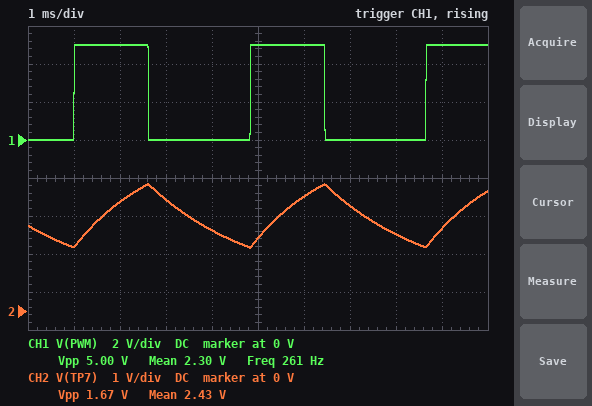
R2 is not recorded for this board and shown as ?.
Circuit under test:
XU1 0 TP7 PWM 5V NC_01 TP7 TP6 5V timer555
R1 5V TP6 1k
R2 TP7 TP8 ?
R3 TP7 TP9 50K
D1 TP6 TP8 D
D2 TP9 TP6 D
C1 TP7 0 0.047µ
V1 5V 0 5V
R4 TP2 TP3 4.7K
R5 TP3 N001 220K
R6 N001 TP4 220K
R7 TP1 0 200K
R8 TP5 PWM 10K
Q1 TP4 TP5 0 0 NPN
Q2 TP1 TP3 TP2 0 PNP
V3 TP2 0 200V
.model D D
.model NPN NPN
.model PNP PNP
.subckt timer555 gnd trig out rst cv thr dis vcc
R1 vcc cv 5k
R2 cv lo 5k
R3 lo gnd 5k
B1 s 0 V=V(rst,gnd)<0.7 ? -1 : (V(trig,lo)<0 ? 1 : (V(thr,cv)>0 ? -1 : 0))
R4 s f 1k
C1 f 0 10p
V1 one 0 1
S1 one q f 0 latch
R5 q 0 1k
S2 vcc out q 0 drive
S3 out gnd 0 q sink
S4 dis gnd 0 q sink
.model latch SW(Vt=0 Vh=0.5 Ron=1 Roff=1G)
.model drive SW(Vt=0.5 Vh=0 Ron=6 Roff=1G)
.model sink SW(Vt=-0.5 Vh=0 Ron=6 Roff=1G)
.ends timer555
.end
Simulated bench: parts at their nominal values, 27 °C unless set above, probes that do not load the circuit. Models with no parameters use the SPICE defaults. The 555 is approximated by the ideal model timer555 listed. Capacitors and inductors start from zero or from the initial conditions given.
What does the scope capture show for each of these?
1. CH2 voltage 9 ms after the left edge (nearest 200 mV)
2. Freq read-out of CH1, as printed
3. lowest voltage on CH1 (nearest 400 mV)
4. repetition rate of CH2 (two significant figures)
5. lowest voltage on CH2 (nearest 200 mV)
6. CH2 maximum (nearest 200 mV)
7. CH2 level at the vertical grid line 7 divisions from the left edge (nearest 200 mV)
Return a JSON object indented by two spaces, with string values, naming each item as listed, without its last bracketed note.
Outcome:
{
  "CH2 voltage 9 ms after the left edge": "2.2 V",
  "Freq read-out of CH1, as printed": "261 Hz",
  "lowest voltage on CH1": "0 V",
  "repetition rate of CH2": "260 Hz",
  "lowest voltage on CH2": "1.6 V",
  "CH2 maximum": "3.4 V",
  "CH2 level at the vertical grid line 7 divisions from the left edge": "2.8 V"
}
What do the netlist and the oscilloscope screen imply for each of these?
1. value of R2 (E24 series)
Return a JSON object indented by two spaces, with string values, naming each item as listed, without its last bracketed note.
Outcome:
{
  "value of R2": "36 kΩ"
}
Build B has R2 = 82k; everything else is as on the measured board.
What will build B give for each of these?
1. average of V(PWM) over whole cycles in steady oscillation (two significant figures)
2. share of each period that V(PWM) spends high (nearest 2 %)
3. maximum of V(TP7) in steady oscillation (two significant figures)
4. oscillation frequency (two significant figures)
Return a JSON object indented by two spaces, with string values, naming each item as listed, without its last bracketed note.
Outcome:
{
  "average of V(PWM) over whole cycles in steady oscillation": "3.1 V",
  "share of each period that V(PWM) spends high": "62 %",
  "maximum of V(TP7) in steady oscillation": "3.3 V",
  "oscillation frequency": "170 Hz"
}
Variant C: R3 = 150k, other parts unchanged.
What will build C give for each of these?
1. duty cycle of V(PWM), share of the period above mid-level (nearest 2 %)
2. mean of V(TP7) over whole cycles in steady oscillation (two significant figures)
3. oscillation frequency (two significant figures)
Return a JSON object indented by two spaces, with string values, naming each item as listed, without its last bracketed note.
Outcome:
{
  "duty cycle of V(PWM), share of the period above mid-level": "20 %",
  "mean of V(TP7) over whole cycles in steady oscillation": "2.4 V",
  "oscillation frequency": "120 Hz"
}
